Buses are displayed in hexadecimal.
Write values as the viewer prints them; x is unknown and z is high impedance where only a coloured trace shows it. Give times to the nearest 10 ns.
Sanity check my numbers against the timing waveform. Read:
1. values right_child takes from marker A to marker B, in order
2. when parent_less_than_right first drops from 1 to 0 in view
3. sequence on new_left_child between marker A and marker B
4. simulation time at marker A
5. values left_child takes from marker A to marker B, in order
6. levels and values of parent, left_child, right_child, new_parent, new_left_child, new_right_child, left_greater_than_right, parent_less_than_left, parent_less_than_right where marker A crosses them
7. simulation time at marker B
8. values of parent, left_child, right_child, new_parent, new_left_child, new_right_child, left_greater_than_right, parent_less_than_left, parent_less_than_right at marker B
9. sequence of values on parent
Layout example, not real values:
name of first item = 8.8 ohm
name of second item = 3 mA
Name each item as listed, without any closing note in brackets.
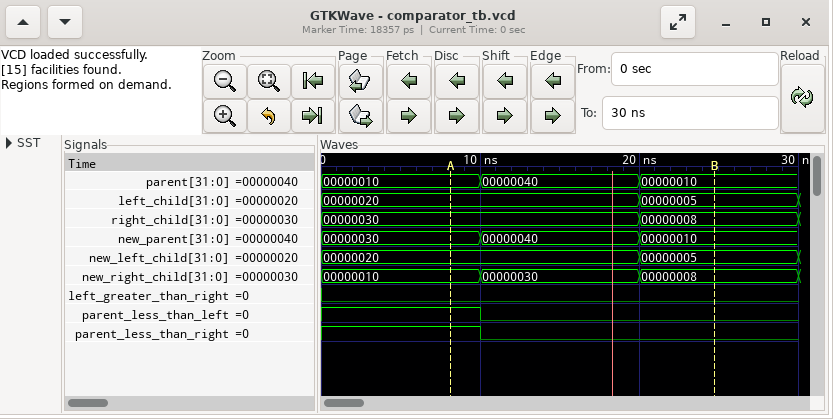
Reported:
values right_child takes from marker A to marker B, in order = 00000030, 00000008
when parent_less_than_right first drops from 1 to 0 in view = 10 ns
sequence on new_left_child between marker A and marker B = 00000020, 00000005
simulation time at marker A = 10 ns
values left_child takes from marker A to marker B, in order = 00000020, 00000005
levels and values of parent, left_child, right_child, new_parent, new_left_child, new_right_child, left_greater_than_right, parent_less_than_left, parent_less_than_right where marker A crosses them = parent=00000010, left_child=00000020, right_child=00000030, new_parent=00000030, new_left_child=00000020, new_right_child=00000010, left_greater_than_right=0, parent_less_than_left=1, parent_less_than_right=1
simulation time at marker B = 20 ns
values of parent, left_child, right_child, new_parent, new_left_child, new_right_child, left_greater_than_right, parent_less_than_left, parent_less_than_right at marker B = parent=00000010, left_child=00000005, right_child=00000008, new_parent=00000010, new_left_child=00000005, new_right_child=00000008, left_greater_than_right=0, parent_less_than_left=0, parent_less_than_right=0
sequence of values on parent = 00000010, 00000040, 00000010
